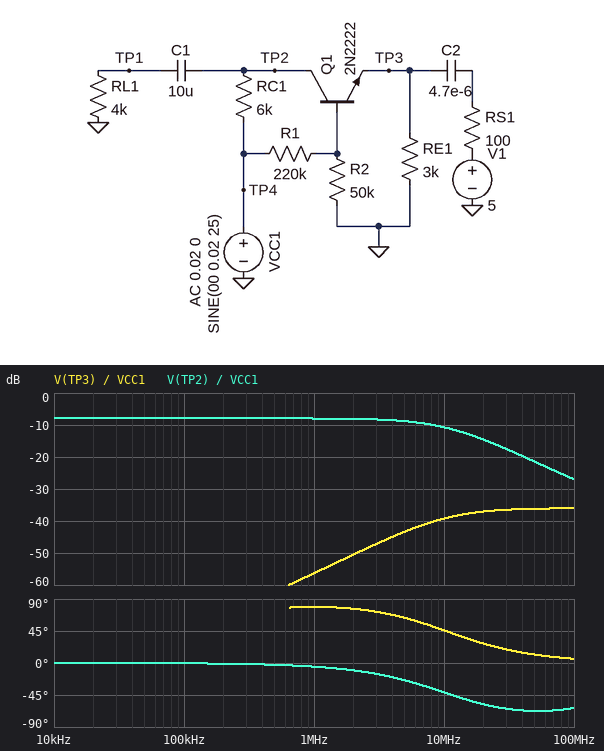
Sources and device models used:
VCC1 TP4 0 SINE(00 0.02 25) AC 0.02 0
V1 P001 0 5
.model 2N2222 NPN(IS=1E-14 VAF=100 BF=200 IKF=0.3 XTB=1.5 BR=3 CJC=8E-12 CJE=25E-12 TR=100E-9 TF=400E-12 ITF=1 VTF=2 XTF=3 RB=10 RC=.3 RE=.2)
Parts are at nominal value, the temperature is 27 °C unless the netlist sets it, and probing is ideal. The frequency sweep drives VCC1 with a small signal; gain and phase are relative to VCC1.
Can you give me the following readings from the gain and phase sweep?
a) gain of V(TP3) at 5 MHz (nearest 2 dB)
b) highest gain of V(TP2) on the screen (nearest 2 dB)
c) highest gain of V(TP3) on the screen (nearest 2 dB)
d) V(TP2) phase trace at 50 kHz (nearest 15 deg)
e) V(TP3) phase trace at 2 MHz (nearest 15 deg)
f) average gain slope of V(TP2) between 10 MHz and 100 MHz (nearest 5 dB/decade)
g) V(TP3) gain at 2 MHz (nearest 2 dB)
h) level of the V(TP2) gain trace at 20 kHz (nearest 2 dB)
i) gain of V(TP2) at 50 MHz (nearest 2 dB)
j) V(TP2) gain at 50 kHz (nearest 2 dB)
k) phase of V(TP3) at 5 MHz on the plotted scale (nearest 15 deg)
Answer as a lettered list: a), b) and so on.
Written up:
a) -44 dB
b) -8 dB
c) -36 dB
d) 0 deg
e) 75 deg
f) -15 dB/decade
g) -50 dB
h) -8 dB
i) -22 dB
j) -8 dB
k) 60 deg
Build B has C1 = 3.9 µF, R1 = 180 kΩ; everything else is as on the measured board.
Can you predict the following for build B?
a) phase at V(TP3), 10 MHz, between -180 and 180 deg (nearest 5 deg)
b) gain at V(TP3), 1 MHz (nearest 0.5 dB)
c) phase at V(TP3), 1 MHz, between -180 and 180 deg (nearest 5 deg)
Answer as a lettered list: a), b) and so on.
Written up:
a) 45 deg
b) -56.0 dB
c) 75 deg
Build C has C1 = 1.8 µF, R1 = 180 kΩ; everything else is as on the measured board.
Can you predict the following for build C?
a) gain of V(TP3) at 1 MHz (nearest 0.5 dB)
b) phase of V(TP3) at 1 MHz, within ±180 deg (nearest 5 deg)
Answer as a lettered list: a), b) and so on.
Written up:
a) -56.0 dB
b) 75 deg
